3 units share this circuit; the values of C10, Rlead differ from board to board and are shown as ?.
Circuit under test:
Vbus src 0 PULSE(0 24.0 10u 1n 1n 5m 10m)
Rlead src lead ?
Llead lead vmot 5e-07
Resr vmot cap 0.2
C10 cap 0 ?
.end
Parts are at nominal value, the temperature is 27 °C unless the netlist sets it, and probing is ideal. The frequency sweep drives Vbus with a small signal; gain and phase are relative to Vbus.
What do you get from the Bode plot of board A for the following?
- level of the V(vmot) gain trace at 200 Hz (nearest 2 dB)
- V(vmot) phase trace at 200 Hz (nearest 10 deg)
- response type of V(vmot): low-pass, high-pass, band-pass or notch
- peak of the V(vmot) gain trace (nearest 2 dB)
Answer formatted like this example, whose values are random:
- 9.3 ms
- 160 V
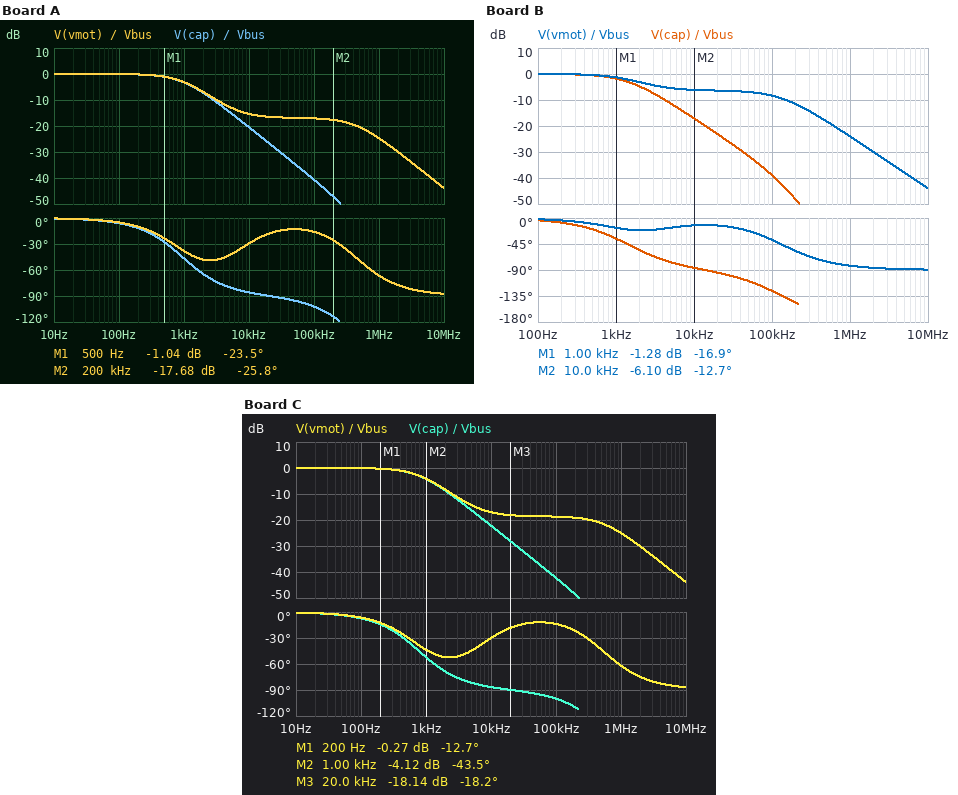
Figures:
- 0 dB
- -10 deg
- low-pass
- 0 dB
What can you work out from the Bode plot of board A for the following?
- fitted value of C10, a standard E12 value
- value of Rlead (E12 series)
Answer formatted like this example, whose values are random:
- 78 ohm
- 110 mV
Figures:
- 120 µF
- 1.2 Ω
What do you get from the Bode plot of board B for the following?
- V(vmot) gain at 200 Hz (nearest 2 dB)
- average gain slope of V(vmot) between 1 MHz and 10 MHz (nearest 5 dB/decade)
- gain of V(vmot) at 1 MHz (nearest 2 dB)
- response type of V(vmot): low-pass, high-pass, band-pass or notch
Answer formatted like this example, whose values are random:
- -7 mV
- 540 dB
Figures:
- 0 dB
- -20 dB/decade
- -24 dB
- low-pass
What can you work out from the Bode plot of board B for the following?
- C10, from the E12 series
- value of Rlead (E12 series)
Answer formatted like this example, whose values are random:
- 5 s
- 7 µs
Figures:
- 270 µF
- 0.22 Ω
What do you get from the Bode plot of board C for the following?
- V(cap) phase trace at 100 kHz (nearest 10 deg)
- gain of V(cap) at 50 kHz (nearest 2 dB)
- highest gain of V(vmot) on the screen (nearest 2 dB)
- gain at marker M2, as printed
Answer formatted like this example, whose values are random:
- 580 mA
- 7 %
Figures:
- -100 deg
- -36 dB
- 0 dB
- -4.12 dB
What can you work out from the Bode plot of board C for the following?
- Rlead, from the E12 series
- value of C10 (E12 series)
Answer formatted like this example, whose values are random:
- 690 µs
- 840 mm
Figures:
- 1.5 Ω
- 120 µF
